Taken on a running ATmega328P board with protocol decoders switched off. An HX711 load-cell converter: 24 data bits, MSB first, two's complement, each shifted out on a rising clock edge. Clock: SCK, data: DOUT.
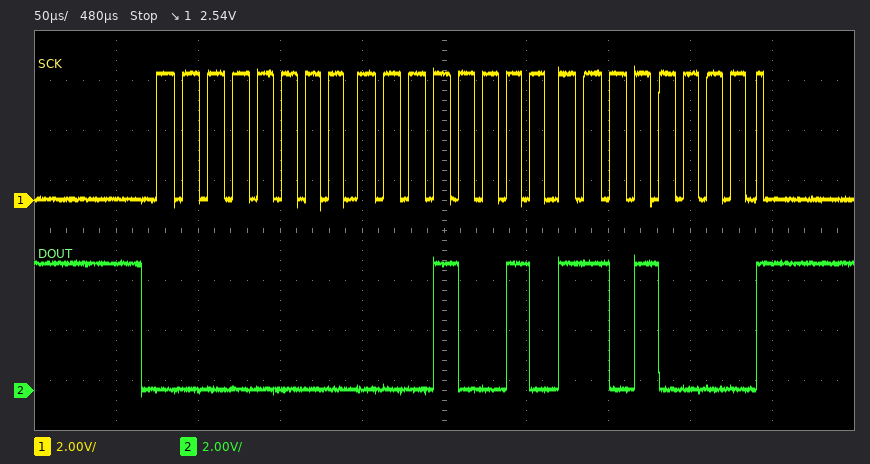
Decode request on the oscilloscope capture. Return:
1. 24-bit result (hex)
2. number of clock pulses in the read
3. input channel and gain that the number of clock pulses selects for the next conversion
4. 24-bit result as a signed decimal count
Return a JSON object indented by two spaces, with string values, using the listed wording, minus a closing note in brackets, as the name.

{
  "24-bit result": "0x0012D0",
  "number of clock pulses in the read": "25",
  "input channel and gain that the number of clock pulses selects for the next conversion": "channel A, gain 128",
  "24-bit result as a signed decimal count": "4816"
}
